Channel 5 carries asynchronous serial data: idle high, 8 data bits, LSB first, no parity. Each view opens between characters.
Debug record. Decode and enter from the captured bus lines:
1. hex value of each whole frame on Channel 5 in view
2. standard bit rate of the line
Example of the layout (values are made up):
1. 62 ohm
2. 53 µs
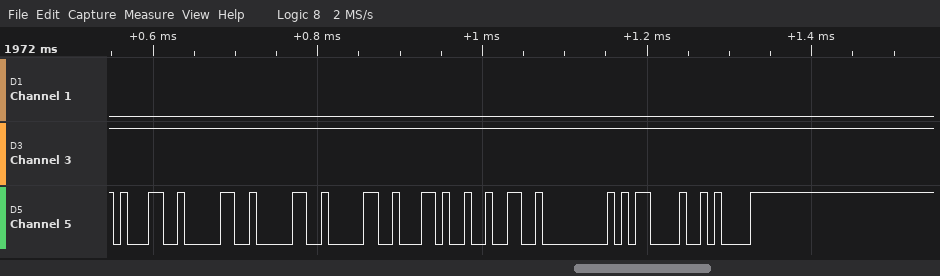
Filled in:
1. 31, 30, 30, 30, 2C, 32, 00, 0D, 0A
2. 115200 baud
